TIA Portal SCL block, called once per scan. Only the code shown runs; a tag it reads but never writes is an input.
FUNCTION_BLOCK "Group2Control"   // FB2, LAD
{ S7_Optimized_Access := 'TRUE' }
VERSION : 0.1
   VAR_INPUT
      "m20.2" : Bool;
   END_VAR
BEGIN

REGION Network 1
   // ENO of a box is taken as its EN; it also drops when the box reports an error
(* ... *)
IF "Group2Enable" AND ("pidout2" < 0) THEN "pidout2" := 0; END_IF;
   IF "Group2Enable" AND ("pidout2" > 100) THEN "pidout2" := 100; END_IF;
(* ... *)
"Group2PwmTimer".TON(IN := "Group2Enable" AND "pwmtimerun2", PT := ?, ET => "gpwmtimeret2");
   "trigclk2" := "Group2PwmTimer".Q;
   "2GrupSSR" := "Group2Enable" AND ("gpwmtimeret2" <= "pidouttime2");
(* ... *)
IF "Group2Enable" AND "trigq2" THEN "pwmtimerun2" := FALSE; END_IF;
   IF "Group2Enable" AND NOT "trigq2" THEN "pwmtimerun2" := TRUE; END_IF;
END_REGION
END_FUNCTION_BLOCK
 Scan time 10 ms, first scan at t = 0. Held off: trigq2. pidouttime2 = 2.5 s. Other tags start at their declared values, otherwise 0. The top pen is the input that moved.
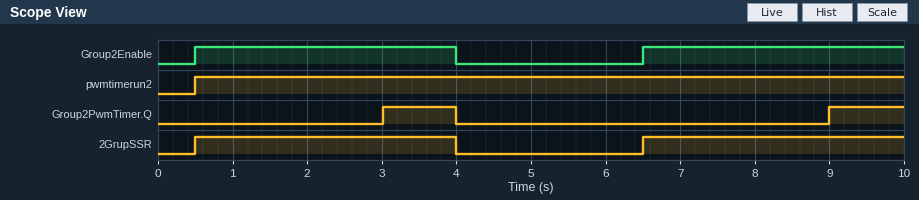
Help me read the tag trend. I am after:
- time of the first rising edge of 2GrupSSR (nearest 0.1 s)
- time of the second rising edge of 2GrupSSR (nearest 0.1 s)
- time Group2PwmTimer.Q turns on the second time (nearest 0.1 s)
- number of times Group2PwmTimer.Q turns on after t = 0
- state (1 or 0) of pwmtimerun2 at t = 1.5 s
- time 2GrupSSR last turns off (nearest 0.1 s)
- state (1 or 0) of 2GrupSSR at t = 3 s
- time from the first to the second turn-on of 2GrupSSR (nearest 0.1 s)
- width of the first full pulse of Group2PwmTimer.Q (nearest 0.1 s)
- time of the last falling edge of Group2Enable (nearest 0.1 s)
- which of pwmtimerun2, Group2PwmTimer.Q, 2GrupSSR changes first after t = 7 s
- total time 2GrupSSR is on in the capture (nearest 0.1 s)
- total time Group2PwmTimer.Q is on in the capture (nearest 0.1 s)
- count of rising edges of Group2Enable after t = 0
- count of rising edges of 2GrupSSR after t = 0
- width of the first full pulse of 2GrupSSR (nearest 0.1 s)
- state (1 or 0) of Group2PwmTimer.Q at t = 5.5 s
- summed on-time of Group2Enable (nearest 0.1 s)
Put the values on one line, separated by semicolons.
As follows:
0.5 s; 6.5 s; 9.0 s; 2; 1; 4.0 s; 1; 6.0 s; 1.0 s; 4.0 s; Group2PwmTimer.Q; 7.0 s; 2.0 s; 2; 2; 3.5 s; 0; 7.0 s
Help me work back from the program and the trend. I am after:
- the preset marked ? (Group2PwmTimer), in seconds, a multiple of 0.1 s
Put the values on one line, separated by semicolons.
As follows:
2.5 s
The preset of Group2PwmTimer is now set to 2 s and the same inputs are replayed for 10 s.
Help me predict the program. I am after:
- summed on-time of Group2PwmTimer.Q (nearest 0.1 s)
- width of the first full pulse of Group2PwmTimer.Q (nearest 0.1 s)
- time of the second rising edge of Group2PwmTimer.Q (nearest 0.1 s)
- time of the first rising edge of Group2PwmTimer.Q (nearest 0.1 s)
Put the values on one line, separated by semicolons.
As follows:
3.0 s; 1.5 s; 8.5 s; 2.5 s
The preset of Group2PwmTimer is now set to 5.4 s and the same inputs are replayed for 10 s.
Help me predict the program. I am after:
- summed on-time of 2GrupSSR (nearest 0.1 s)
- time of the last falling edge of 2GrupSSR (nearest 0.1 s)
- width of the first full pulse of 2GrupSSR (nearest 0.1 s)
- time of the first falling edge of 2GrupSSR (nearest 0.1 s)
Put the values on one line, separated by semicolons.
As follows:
5.0 s; 9.0 s; 2.5 s; 3.0 s
